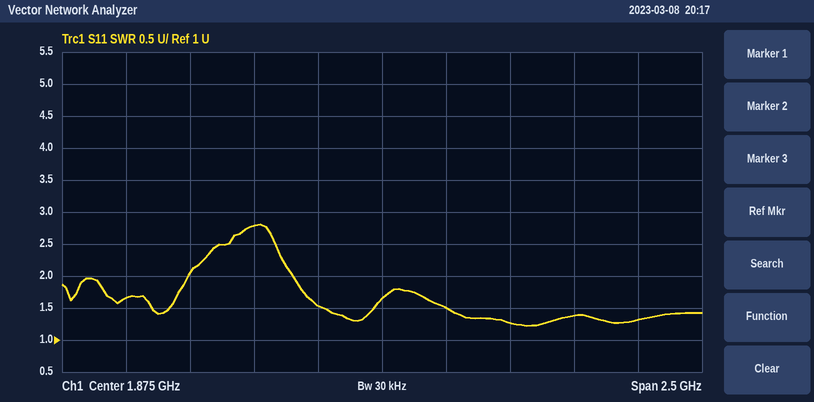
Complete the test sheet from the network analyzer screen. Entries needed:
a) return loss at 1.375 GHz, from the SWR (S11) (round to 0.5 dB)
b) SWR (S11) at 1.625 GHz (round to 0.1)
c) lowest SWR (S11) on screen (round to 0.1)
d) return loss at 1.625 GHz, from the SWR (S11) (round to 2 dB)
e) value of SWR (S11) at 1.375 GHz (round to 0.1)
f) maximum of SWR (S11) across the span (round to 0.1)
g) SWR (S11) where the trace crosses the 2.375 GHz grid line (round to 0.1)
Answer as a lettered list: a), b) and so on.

a) 6.5 dB
b) 1.5
c) 1.2
d) 14 dB
e) 2.8
f) 2.8
g) 1.3
